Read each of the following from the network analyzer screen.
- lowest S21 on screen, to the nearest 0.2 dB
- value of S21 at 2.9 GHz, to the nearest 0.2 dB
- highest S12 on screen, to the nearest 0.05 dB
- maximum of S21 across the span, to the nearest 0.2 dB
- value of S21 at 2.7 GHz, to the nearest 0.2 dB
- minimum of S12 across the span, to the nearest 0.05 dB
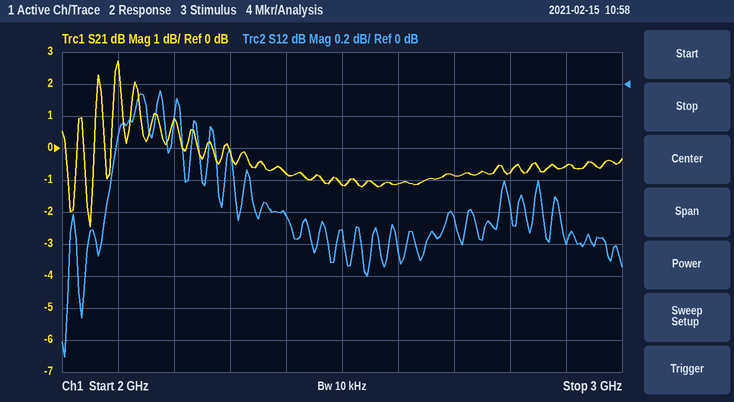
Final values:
-2.4 dB
-0.6 dB
-0.05 dB
2.8 dB
-0.8 dB
-1.70 dB
